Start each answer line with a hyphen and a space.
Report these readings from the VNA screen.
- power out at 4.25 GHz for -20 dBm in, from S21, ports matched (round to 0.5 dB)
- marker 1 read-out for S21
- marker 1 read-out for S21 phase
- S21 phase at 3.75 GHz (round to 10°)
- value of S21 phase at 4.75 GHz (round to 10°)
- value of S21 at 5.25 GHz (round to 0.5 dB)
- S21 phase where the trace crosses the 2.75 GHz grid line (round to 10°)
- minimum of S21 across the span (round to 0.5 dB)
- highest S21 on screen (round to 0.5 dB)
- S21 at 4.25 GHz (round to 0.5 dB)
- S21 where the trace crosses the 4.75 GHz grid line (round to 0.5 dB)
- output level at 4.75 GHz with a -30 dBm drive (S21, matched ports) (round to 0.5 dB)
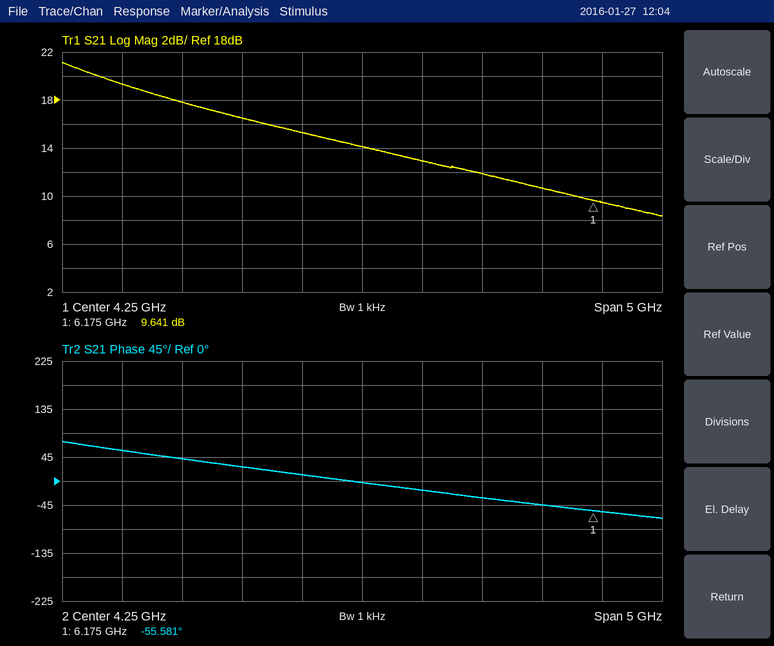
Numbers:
- -6.0 dBm
- 9.641 dB
- -55.581°
- 10°
- -20°
- 12.0 dB
- 40°
- 8.5 dB
- 21.0 dB
- 14.0 dB
- 13.0 dB
- -17.0 dBm
